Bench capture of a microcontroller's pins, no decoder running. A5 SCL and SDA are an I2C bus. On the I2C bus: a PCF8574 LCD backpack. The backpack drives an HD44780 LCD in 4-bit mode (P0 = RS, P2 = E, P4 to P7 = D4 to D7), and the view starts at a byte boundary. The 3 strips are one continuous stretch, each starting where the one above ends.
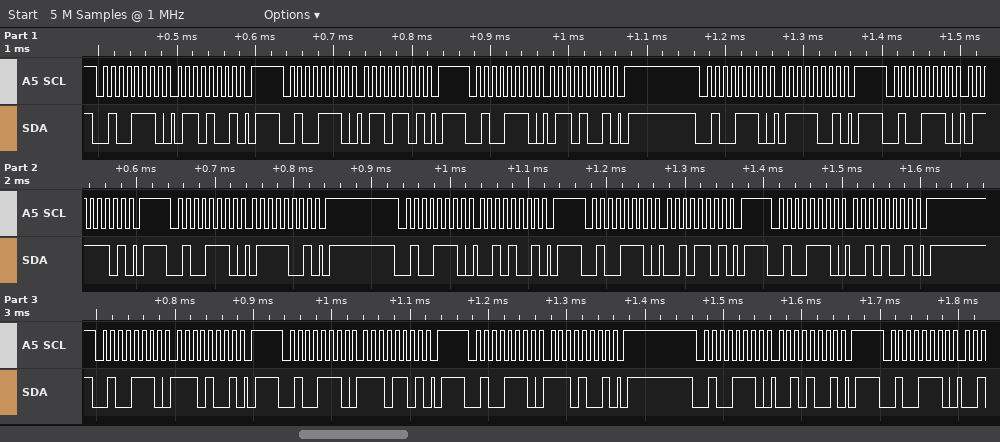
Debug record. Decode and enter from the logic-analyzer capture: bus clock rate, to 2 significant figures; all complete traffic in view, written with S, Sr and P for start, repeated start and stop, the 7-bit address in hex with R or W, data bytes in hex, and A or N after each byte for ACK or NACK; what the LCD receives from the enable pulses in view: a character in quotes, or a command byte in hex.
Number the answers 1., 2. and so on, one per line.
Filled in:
1. 100 kHz
2. S 27W A 69 A P S 27W A 6D A P S 27W A 69 A P S 27W A 79 A P S 27W A 7D A P S 27W A 79 A P S 27W A 29 A P S 27W A 2D A P S 27W A 29 A P S 27W A E9 A P S 27W A ED A P S 27W A E9 A P S 27W A 29 A P S 27W A
3. 'g' '.'
